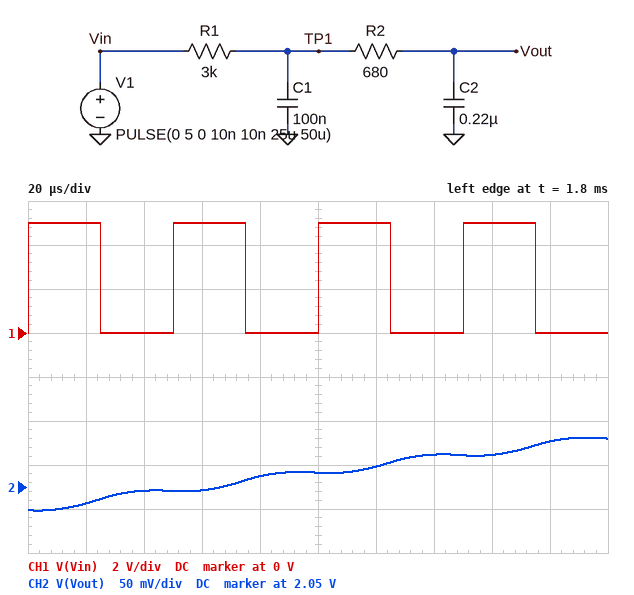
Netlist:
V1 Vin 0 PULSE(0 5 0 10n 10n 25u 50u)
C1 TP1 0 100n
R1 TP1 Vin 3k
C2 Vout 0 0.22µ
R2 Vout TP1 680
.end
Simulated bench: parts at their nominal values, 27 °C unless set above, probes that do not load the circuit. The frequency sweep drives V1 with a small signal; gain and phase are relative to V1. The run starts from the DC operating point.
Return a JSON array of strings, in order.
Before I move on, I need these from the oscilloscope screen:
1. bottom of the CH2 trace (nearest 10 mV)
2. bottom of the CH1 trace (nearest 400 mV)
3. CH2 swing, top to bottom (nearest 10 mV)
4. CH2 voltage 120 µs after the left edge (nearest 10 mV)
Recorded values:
["2.02 V", "0 V", "80 mV", "2.07 V"]
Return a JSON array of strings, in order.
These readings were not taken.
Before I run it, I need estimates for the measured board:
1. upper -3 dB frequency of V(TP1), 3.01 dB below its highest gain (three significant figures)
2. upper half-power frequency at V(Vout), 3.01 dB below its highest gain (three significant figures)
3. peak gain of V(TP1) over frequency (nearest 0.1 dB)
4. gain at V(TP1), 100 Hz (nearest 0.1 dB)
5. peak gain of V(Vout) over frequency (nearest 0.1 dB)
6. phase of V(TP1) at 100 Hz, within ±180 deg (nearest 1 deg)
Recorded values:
["152 Hz", "149 Hz", "0 dB", "-1.6 dB", "0 dB", "-30 deg"]
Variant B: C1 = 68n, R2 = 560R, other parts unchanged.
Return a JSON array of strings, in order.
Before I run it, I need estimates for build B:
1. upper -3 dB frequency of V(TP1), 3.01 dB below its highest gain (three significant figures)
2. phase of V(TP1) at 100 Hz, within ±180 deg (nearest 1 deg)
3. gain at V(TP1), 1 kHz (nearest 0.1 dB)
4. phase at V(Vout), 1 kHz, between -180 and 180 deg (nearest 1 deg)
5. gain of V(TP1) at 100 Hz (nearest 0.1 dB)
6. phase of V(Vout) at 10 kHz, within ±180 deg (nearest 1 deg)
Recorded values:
["168 Hz", "-28 deg", "-13.8 dB", "-90 deg", "-1.3 dB", "-148 deg"]
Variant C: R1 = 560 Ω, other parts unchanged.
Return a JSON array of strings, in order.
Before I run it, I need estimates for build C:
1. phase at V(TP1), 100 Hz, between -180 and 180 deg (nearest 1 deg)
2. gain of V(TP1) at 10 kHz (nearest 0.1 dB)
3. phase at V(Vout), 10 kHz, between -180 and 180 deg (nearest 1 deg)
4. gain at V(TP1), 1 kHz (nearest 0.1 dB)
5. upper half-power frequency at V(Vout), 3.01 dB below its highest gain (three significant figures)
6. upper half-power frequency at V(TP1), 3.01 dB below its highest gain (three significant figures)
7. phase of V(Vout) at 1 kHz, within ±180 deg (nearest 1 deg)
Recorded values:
["-6 deg", "-12.1 dB", "-147 deg", "-4.0 dB", "524 Hz", "726 Hz", "-72 deg"]
